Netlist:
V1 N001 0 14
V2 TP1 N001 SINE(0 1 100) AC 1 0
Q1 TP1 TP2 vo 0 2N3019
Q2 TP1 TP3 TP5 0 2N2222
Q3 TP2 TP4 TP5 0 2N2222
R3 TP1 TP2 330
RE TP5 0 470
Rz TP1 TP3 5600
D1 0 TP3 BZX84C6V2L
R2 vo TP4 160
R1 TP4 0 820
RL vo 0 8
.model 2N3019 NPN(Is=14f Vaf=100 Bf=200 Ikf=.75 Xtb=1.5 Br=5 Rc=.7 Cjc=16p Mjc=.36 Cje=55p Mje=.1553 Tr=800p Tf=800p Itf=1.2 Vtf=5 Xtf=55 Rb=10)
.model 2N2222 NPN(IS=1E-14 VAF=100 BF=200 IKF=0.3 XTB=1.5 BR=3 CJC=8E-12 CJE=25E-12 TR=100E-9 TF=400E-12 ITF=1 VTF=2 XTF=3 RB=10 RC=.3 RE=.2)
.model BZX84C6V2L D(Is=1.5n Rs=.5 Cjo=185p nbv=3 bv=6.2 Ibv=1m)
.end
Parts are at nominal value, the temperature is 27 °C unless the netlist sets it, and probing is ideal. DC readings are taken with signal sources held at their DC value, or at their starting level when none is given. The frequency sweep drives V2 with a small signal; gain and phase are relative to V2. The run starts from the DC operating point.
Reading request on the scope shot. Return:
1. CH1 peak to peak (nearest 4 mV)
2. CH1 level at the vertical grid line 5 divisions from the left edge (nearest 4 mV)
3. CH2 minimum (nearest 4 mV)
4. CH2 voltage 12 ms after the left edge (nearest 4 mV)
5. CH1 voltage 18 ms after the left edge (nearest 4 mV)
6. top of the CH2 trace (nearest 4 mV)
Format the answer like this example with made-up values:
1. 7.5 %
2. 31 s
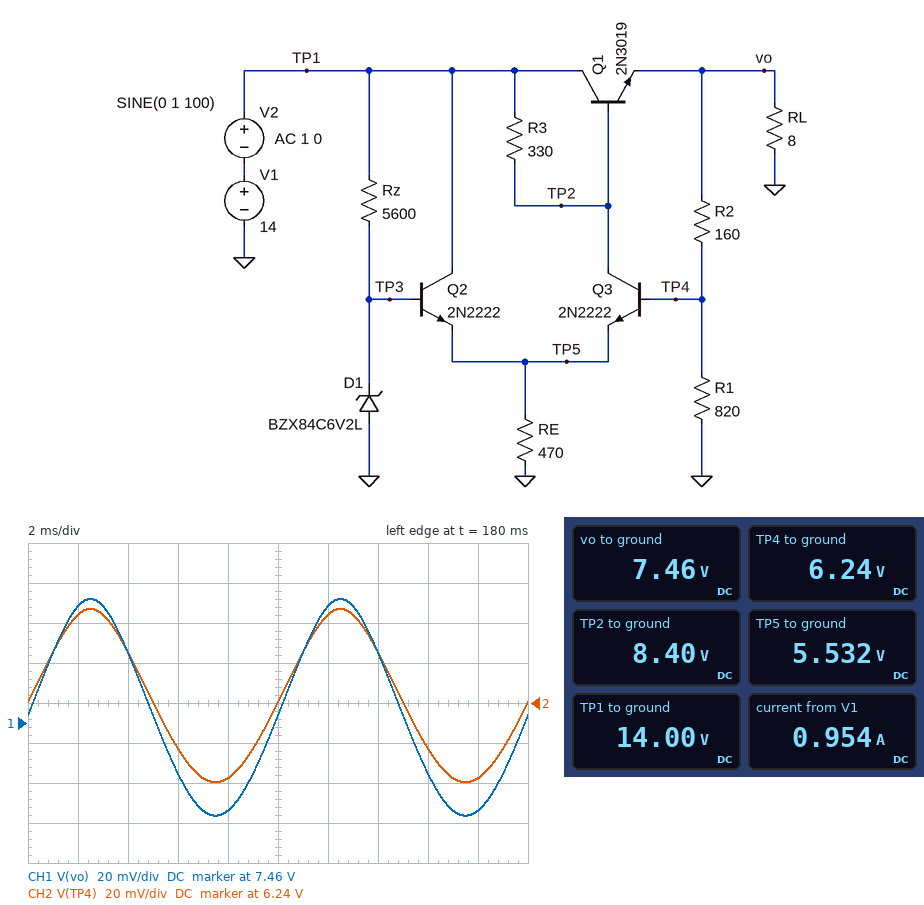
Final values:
1. 108 mV
2. 7.464 V
3. 6.200 V
4. 6.284 V
5. 7.416 V
6. 6.288 V
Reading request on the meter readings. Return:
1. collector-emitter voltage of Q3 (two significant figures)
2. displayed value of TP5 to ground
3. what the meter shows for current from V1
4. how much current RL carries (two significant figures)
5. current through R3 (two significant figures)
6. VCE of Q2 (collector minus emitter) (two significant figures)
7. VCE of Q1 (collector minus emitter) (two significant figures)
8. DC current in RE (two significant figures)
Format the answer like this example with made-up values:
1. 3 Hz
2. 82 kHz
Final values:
1. 2.9 V
2. 5.532 V
3. 0.954 A
4. 930 mA
5. 17 mA
6. 8.5 V
7. 6.5 V
8. 12 mA
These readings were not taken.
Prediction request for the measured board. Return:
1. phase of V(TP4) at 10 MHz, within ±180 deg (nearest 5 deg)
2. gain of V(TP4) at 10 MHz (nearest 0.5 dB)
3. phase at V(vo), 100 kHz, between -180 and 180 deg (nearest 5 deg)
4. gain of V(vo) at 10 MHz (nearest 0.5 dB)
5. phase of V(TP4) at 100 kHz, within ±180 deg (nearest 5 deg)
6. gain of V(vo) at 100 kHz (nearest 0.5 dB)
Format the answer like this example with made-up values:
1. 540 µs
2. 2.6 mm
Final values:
1. 0 deg
2. -14.5 dB
3. 10 deg
4. -11.0 dB
5. 10 deg
6. -26.0 dB
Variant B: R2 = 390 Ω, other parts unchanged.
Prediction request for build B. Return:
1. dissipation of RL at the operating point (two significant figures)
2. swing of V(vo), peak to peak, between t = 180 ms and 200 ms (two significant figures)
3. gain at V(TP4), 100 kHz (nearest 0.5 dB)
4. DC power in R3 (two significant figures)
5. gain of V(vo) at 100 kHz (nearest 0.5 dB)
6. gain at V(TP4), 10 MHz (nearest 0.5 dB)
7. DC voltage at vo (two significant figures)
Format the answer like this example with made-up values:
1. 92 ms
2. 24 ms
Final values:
1. 9.7 W
2. 890 mV
3. -9.0 dB
4. 54 mW
5. -5.5 dB
6. -13.5 dB
7. 8.8 V
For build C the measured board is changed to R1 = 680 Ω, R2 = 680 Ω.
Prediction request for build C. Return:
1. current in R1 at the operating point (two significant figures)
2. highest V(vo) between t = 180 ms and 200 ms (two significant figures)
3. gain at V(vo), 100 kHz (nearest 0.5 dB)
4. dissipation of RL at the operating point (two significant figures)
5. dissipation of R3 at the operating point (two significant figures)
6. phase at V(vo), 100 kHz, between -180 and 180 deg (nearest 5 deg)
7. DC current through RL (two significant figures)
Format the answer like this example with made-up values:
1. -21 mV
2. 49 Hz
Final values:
1. 6.5 mA
2. 9.4 V
3. -5.5 dB
4. 9.7 W
5. 54 mW
6. -10 deg
7. 1.1 A
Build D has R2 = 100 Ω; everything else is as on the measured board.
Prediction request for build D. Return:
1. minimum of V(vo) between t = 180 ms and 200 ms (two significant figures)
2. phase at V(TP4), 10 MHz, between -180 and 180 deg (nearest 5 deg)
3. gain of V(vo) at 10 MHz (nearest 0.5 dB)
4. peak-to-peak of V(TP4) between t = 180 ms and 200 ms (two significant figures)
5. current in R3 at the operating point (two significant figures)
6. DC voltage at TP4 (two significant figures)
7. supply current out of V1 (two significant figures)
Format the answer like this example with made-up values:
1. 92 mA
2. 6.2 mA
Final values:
1. 7.0 V
2. 5 deg
3. -11.5 dB
4. 170 mV
5. 18 mA
6. 6.3 V
7. 900 mA
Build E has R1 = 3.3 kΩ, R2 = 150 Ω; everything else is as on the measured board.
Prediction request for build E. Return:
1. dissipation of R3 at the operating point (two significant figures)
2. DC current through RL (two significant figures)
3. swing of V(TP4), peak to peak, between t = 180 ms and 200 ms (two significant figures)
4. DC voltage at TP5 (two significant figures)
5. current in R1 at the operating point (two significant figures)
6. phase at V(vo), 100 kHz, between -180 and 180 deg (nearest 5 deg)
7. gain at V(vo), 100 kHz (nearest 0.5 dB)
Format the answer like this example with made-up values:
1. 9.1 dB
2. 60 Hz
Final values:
1. 130 mW
2. 830 mA
3. 480 mV
4. 5.6 V
5. 1.9 mA
6. 0 deg
7. -13.5 dB
